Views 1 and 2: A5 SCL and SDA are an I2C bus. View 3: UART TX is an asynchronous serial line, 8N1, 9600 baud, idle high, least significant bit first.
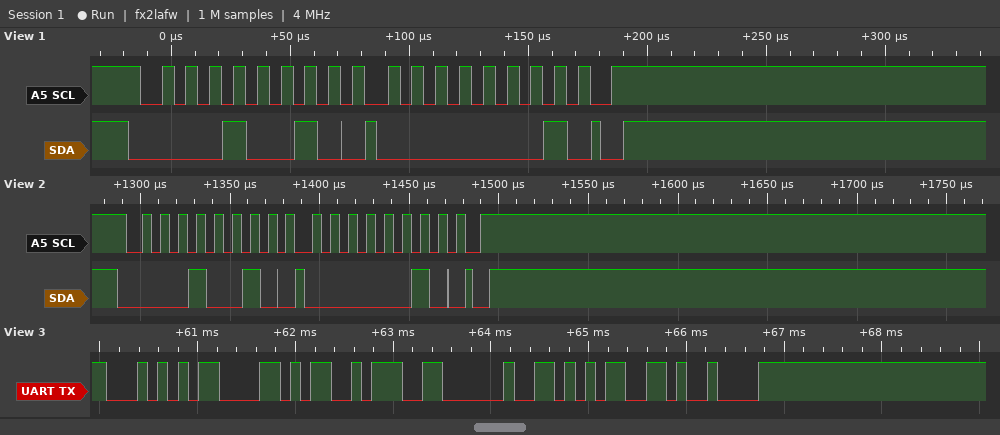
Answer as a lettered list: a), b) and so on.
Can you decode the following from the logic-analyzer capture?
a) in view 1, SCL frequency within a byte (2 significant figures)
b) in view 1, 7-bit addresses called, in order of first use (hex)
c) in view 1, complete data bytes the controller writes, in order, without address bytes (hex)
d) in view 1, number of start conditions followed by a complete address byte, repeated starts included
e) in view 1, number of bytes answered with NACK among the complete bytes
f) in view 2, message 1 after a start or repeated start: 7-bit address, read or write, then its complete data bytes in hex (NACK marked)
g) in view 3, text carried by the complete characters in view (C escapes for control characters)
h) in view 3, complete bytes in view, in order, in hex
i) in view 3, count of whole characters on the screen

a) 100 kHz
b) 0x09
c) 01
d) 1
e) 0
f) 0x09 write: 02
g) "TX: 5\t"
h) 54 58 3A 20 35 09
i) 6
